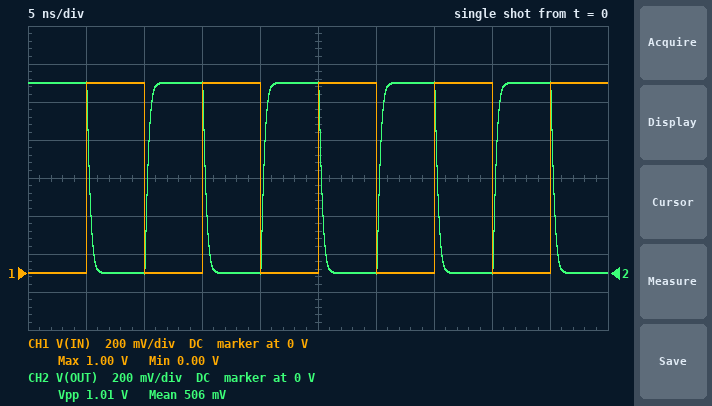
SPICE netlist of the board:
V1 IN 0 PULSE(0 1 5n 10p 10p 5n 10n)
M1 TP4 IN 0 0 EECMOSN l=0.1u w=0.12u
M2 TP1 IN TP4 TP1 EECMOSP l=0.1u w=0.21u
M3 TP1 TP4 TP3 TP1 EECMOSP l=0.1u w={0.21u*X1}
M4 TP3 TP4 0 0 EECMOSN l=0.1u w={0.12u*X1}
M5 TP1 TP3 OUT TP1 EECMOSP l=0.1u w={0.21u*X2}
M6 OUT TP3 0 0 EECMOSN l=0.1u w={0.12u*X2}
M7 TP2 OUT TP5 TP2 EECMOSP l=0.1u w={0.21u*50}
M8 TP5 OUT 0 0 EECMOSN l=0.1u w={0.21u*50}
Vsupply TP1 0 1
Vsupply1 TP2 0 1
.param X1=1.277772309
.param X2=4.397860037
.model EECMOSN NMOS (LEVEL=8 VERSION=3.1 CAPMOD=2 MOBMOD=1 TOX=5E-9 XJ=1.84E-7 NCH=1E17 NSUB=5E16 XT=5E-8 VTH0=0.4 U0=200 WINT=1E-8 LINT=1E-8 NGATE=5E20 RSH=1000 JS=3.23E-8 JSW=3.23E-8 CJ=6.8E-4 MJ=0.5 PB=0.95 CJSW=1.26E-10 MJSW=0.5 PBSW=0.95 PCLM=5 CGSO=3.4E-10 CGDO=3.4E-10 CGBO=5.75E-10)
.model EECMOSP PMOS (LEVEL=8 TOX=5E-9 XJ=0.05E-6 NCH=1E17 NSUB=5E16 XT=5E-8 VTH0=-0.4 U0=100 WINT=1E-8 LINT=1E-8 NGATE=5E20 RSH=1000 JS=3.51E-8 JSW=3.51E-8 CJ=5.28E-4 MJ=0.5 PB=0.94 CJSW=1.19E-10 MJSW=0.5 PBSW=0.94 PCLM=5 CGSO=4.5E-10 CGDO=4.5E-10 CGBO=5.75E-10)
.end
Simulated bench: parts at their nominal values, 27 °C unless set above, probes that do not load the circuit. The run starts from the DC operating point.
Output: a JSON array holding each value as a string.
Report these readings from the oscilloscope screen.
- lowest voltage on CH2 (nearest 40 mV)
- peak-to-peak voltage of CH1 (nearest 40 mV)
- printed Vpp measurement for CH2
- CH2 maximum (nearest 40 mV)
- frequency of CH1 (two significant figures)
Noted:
["0 V", "1.00 V", "1.01 V", "1.00 V", "100 MHz"]
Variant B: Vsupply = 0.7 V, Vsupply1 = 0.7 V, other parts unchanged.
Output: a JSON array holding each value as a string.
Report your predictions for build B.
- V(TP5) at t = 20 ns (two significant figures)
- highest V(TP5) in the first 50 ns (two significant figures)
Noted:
["690 mV", "710 mV"]
